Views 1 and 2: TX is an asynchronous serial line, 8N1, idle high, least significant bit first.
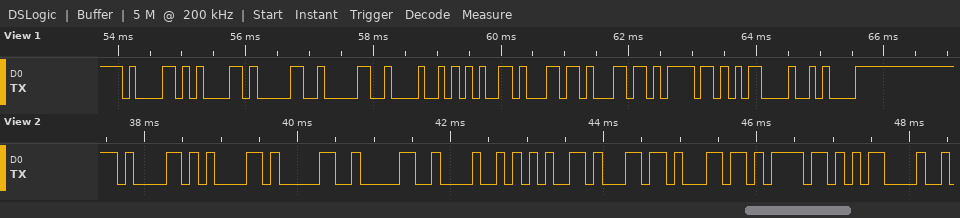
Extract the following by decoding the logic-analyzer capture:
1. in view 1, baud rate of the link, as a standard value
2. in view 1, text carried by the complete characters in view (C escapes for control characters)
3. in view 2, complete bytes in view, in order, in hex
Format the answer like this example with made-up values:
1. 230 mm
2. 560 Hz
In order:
1. 9600 baud
2. "aa00Hello\r\n"
3. 61 61 30 30 48 65 6C 6C 6F 0D
